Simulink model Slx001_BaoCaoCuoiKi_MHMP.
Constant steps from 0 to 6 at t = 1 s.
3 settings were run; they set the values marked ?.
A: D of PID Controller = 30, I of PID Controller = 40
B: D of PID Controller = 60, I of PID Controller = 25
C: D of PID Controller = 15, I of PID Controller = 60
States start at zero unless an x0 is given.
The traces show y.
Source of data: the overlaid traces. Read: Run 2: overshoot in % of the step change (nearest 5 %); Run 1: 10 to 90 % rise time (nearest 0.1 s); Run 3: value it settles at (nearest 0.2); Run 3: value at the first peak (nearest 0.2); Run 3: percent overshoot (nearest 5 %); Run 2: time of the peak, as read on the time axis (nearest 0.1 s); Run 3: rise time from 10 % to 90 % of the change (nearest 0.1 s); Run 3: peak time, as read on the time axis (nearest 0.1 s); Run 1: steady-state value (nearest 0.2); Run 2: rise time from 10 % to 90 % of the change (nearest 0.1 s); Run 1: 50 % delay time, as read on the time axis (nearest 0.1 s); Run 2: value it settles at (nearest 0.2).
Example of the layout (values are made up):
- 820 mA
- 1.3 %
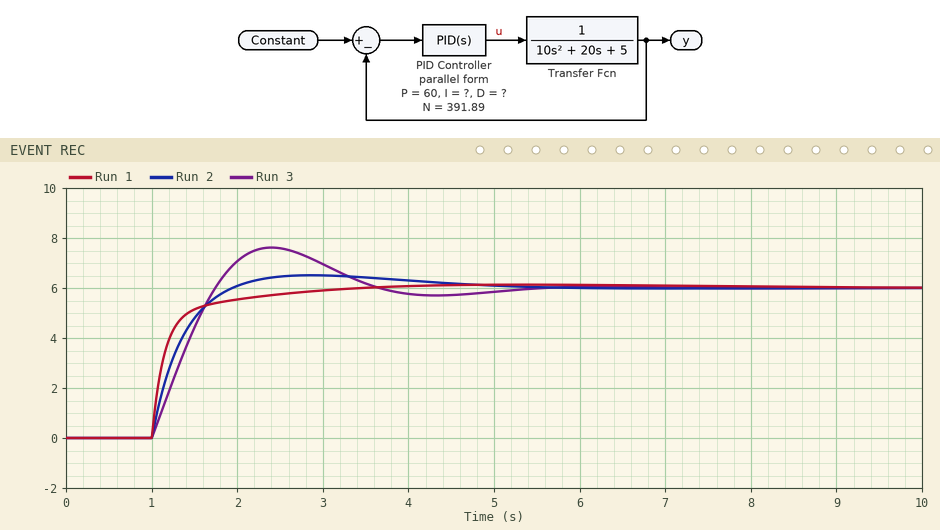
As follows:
- 10 %
- 0.7 s
- 6.0
- 7.6
- 25 %
- 2.9 s
- 0.6 s
- 2.4 s
- 6.0
- 0.6 s
- 1.1 s
- 6.0
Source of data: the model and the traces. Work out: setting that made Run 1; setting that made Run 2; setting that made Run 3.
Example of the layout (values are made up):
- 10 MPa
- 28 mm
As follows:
- B
- A
- C
